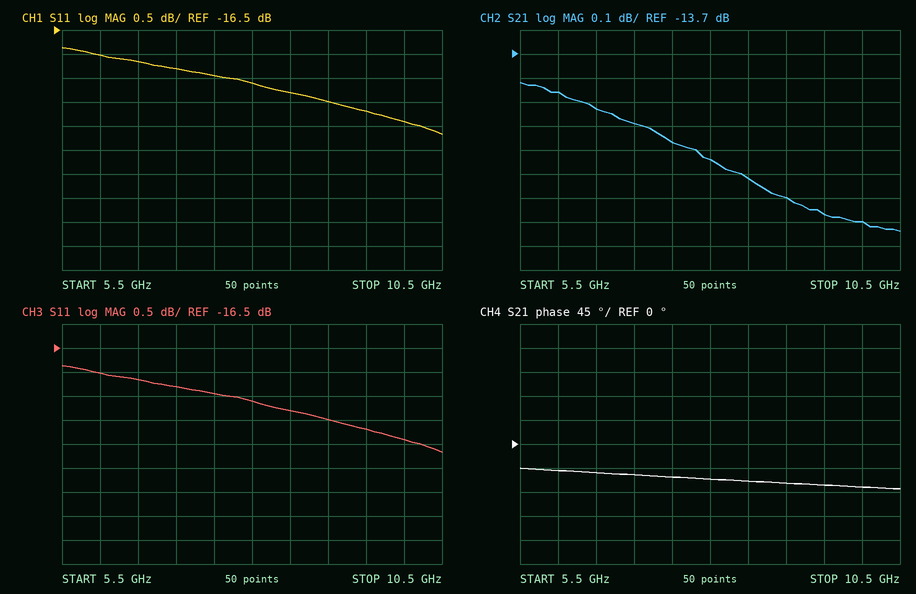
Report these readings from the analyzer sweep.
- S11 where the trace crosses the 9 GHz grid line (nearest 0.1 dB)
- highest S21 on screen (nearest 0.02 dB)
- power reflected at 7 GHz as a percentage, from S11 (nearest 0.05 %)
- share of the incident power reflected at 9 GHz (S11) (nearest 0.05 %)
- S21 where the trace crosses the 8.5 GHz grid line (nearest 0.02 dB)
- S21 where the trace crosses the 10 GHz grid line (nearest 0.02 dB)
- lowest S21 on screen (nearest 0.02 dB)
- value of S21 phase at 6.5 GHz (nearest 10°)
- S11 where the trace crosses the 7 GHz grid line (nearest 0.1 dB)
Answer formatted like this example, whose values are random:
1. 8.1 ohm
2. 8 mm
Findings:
1. -18.0 dB
2. -13.82 dB
3. 1.85 %
4. 1.60 %
5. -14.22 dB
6. -14.40 dB
7. -14.44 dB
8. -50°
9. -17.3 dB
